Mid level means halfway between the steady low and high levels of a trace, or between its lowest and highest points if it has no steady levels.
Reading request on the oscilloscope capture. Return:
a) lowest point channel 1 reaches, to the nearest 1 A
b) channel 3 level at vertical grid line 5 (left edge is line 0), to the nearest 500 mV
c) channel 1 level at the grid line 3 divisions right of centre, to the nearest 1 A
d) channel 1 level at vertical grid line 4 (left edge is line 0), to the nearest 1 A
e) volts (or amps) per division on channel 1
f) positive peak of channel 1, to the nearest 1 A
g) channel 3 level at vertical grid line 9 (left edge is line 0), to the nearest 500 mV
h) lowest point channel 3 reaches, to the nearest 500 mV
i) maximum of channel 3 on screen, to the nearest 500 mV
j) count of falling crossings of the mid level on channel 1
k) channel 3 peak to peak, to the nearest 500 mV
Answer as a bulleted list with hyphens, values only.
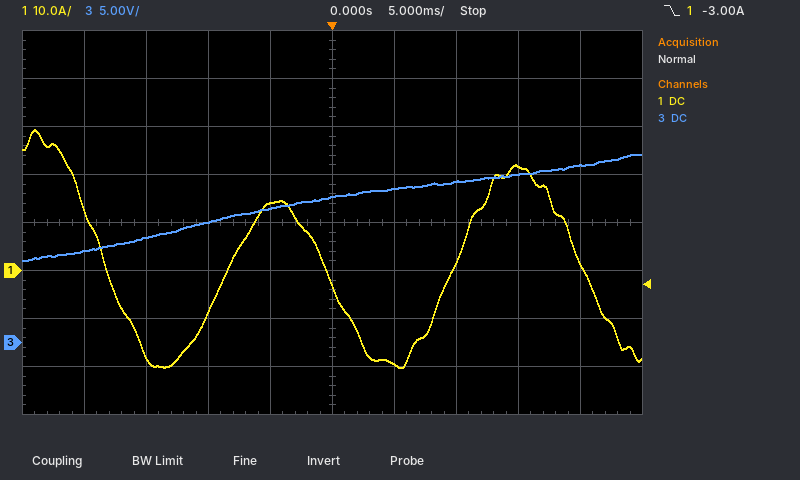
- -20 A
- 15.0 V
- 22 A
- 14 A
- 10 A
- 29 A
- 18.5 V
- 8.5 V
- 19.5 V
- 3
- 11.0 V
